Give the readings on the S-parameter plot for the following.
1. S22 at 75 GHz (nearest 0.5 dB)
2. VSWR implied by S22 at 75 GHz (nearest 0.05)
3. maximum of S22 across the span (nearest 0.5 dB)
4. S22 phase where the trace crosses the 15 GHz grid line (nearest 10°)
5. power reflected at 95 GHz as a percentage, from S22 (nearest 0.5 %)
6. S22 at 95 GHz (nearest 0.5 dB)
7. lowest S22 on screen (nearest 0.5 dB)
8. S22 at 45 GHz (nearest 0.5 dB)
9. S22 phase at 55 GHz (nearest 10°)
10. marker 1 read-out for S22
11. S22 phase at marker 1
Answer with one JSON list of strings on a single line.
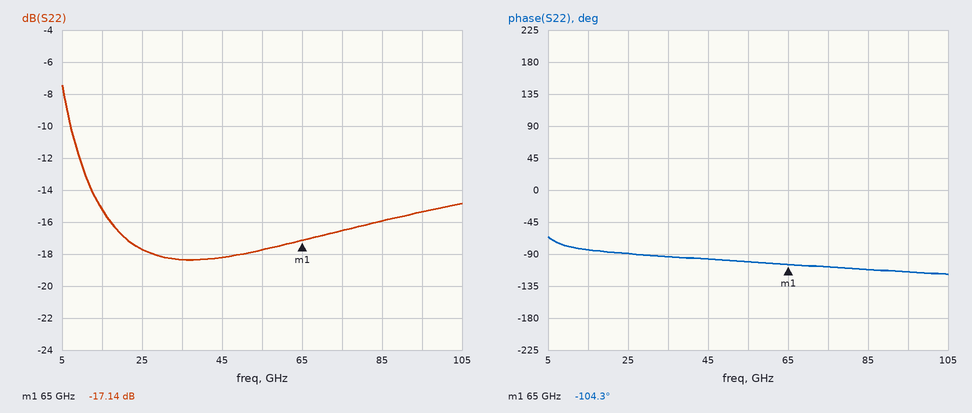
["-16.5 dB", "1.35", "-7.5 dB", "-80°", "3.0 %", "-15.5 dB", "-18.5 dB", "-18.0 dB", "-100°", "-17.14 dB", "-104.3°"]
